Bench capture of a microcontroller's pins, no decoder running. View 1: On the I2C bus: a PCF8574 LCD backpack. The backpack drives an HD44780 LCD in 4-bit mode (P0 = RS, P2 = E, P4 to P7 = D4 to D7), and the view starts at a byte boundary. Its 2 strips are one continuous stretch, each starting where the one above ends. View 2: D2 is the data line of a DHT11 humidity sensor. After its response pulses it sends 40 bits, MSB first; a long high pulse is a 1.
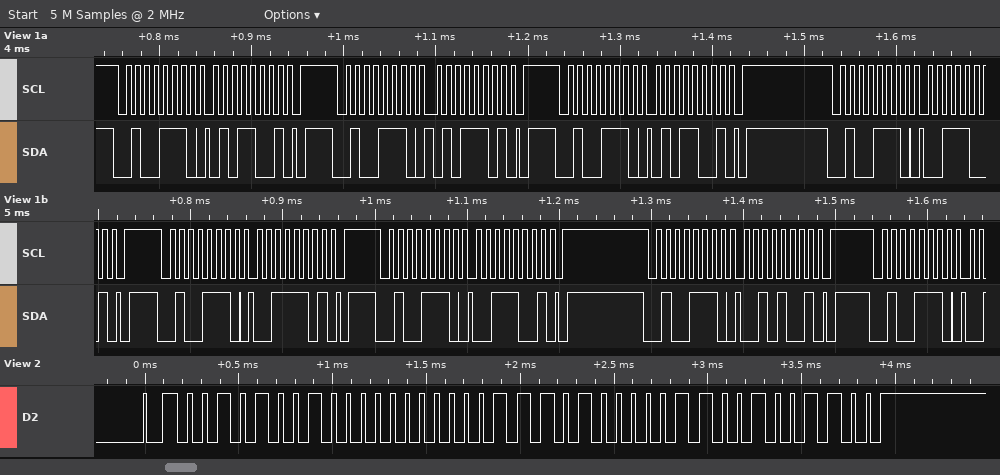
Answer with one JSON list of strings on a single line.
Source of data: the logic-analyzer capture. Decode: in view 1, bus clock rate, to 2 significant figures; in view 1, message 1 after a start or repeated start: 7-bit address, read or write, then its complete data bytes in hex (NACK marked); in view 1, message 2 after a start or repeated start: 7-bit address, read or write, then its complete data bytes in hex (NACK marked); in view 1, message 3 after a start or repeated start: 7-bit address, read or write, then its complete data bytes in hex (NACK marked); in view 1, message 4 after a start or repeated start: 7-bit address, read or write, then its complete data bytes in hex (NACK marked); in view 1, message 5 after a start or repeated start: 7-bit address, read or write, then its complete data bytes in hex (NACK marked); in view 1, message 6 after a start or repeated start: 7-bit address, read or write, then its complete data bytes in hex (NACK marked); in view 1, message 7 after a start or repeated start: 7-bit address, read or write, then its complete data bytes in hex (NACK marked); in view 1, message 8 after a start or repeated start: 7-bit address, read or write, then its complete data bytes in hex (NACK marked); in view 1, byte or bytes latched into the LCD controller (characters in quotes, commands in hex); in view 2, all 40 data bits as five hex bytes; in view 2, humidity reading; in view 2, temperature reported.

["100 kHz", "0x27 write: 59", "0x27 write: 5D", "0x27 write: 59", "0x27 write: 39", "0x27 write: 3D", "0x27 write: 39", "0x27 write: 29", "0x27 write", "'S'", "29 00 1D 06 4C", "41 %", "29.6 °C"]
